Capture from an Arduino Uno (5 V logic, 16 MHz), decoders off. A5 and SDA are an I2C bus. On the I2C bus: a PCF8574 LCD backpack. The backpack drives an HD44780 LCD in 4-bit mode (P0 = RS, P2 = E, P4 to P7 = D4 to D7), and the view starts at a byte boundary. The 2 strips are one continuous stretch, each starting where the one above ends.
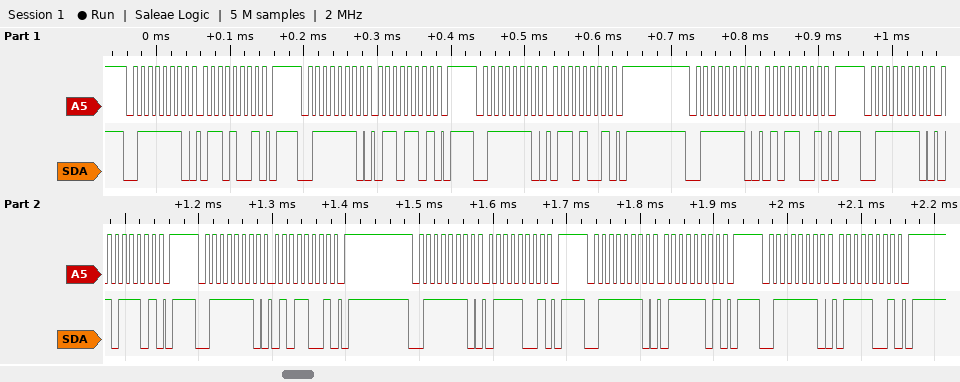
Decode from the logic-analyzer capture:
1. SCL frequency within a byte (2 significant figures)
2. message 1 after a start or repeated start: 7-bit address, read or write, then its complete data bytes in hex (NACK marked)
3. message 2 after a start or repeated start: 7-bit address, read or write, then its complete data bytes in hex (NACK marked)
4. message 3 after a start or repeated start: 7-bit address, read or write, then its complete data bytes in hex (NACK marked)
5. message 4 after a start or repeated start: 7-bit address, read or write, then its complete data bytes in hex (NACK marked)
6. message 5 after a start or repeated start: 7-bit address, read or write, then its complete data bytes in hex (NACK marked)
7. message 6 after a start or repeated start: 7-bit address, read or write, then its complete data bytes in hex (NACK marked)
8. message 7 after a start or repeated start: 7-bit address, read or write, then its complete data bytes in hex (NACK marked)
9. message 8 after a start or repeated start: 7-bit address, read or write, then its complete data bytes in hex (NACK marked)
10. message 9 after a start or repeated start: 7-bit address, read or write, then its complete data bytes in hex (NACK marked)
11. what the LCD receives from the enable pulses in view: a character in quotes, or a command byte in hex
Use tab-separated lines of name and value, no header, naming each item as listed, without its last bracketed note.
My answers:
SCL frequency within a byte	100 kHz
message 1 after a start or repeated start: 7-bit address, read or write, then its complete data bytes in hex	0x3F write: 69
message 2 after a start or repeated start: 7-bit address, read or write, then its complete data bytes in hex	0x3F write: 6D
message 3 after a start or repeated start: 7-bit address, read or write, then its complete data bytes in hex	0x3F write: 69
message 4 after a start or repeated start: 7-bit address, read or write, then its complete data bytes in hex	0x3F write: 59
message 5 after a start or repeated start: 7-bit address, read or write, then its complete data bytes in hex	0x3F write: 5D
message 6 after a start or repeated start: 7-bit address, read or write, then its complete data bytes in hex	0x3F write: 59
message 7 after a start or repeated start: 7-bit address, read or write, then its complete data bytes in hex	0x3F write: 79
message 8 after a start or repeated start: 7-bit address, read or write, then its complete data bytes in hex	0x3F write: 7D
message 9 after a start or repeated start: 7-bit address, read or write, then its complete data bytes in hex	0x3F write: 79
what the LCD receives from the enable pulses in view: a character in quotes, or a command byte in hex	'e'
